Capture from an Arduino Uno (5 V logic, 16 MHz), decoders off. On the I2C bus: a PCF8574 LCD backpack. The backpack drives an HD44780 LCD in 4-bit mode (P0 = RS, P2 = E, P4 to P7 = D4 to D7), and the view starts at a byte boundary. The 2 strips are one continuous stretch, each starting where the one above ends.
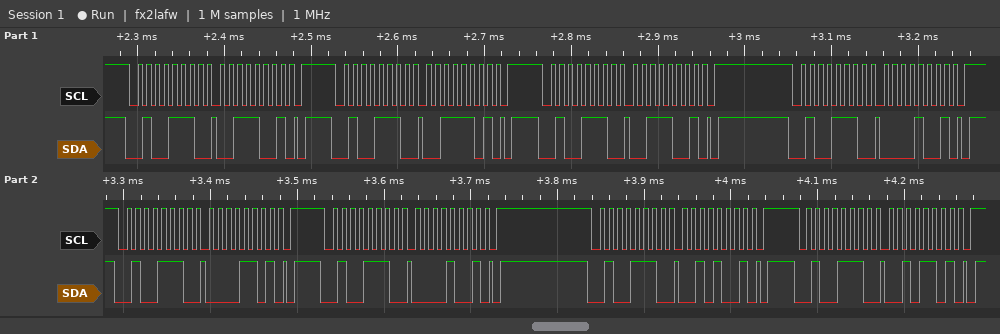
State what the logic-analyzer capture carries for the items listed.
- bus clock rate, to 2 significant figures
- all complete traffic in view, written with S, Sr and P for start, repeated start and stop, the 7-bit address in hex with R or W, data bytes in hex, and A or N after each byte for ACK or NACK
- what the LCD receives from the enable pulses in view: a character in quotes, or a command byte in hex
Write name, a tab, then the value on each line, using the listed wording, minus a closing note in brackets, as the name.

bus clock rate, to 2 significant figures	100 kHz
all complete traffic in view, written with S, Sr and P for start, repeated start and stop, the 7-bit address in hex with R or W, data bytes in hex, and A or N after each byte for ACK or NACK	S 27W A 39 A P S 27W A 3D A P S 27W A 39 A P S 27W A 09 A P S 27W A 0D A P S 27W A 09 A P S 27W A 29 A P S 27W A 2D A P
what the LCD receives from the enable pulses in view: a character in quotes, or a command byte in hex	'0'
